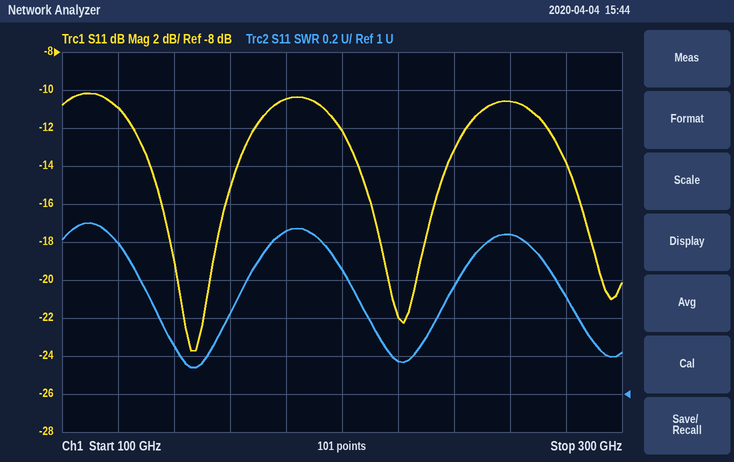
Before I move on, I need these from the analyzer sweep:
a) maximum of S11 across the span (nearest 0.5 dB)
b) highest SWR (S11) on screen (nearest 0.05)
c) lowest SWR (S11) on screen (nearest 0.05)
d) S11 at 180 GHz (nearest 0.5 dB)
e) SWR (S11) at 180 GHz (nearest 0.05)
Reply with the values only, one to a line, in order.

-10.0 dB
1.90
1.15
-10.5 dB
1.85
